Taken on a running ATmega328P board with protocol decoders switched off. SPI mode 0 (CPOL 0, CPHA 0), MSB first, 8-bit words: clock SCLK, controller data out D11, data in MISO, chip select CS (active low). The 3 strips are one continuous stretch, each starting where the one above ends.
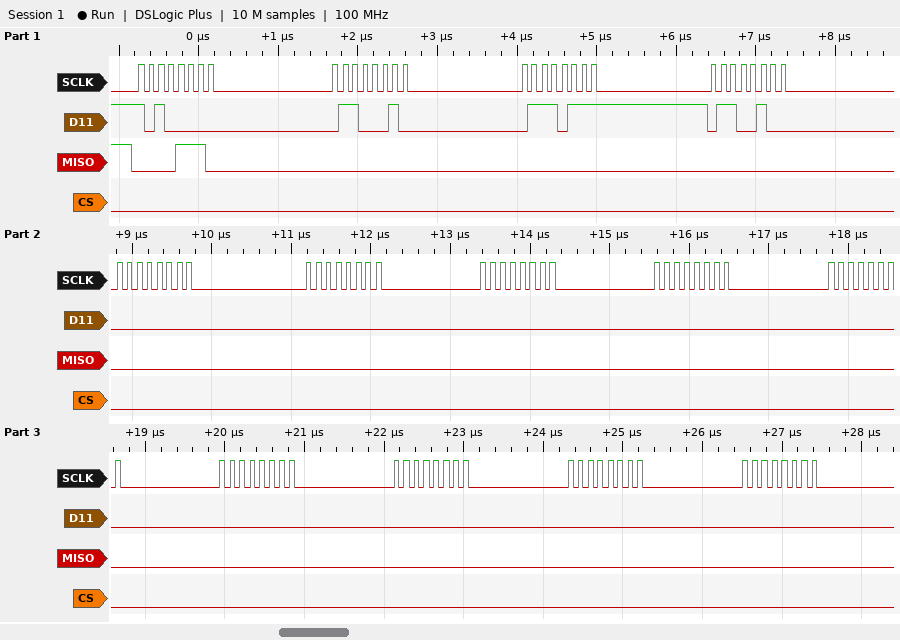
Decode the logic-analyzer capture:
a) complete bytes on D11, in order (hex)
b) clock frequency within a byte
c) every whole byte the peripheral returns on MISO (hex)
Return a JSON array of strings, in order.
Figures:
["A0 62 77 64 00 00 00 00 00 00 00 00 00", "8 MHz", "0E 00 00 00 00 00 00 00 00 00 00 00 00"]
